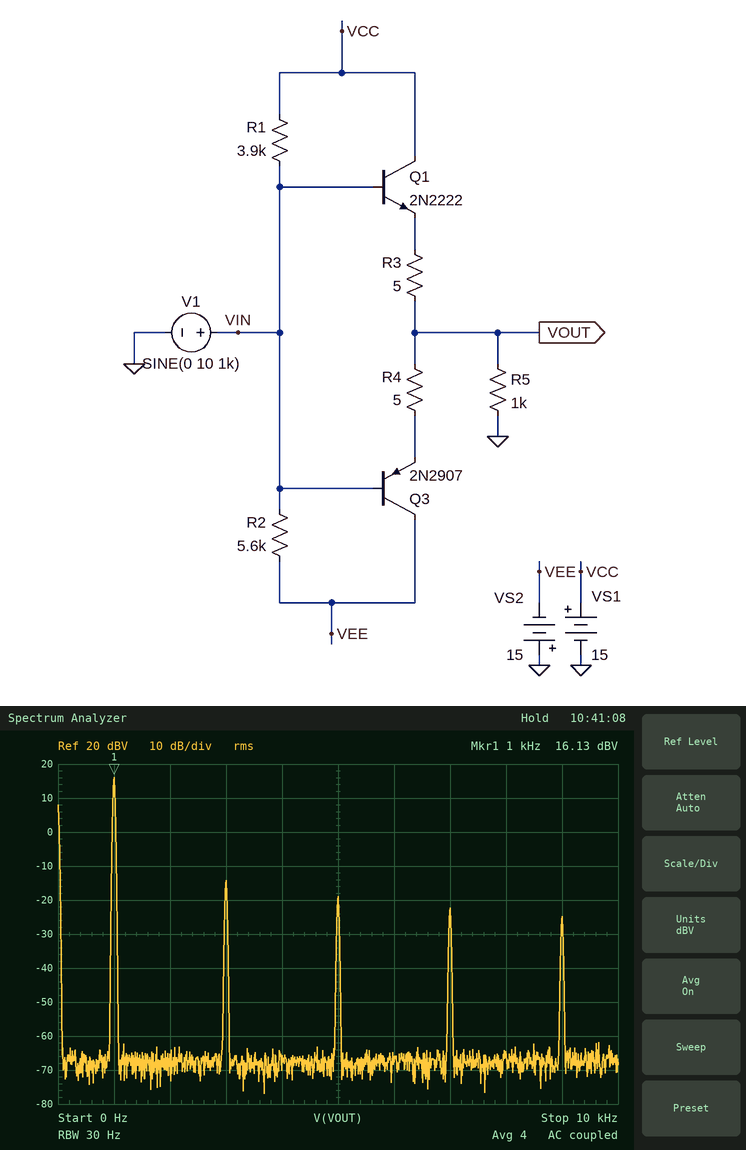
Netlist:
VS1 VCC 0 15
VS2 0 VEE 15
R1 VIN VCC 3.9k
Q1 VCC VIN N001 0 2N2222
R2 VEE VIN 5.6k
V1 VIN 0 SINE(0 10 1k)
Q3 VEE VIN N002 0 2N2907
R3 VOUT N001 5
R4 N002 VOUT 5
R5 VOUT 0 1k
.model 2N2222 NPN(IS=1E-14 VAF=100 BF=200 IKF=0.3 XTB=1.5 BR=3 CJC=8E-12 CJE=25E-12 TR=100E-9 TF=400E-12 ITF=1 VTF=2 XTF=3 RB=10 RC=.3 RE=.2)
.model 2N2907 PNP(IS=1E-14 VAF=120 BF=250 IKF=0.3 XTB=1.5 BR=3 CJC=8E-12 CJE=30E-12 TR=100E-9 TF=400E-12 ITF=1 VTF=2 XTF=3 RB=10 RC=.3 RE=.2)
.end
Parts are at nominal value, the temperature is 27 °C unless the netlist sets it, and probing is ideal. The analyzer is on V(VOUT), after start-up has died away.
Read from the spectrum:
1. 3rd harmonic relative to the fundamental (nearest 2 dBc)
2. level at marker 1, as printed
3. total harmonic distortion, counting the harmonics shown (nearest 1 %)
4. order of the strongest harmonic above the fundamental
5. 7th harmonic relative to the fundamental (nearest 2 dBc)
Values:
-30 dBc
16.13 dBV
4 %
3
-38 dBc
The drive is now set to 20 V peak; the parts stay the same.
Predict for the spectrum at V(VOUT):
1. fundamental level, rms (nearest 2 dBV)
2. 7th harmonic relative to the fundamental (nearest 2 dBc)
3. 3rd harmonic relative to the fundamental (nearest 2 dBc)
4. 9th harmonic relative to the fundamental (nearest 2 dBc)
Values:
22 dBV
-40 dBc
-22 dBc
-44 dBc
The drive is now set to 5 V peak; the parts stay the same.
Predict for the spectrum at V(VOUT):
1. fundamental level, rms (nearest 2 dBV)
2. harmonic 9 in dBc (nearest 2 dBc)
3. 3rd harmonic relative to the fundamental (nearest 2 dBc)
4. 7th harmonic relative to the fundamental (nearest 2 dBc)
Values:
10 dBV
-36 dBc
-24 dBc
-32 dBc
